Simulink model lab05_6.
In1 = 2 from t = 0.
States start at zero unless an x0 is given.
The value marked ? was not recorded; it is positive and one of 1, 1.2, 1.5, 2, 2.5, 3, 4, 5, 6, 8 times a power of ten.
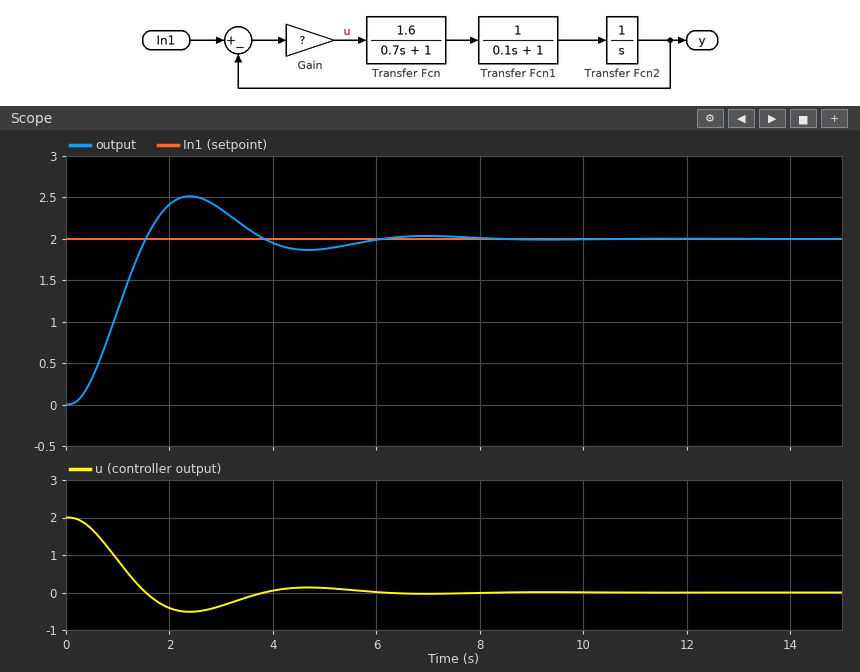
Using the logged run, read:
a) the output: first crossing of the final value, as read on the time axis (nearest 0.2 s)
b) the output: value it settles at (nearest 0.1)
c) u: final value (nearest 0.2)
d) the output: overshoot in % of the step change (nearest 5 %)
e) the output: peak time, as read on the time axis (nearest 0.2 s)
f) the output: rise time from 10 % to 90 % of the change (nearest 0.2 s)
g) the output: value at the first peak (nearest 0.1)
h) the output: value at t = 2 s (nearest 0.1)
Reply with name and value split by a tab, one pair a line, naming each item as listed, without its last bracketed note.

the output: first crossing of the final value, as read on the time axis	1.6 s
the output: value it settles at	2.0
u: final value	0.0
the output: overshoot in % of the step change	25 %
the output: peak time, as read on the time axis	2.4 s
the output: rise time from 10 % to 90 % of the change	1.0 s
the output: value at the first peak	2.5
the output: value at t = 2 s	2.4
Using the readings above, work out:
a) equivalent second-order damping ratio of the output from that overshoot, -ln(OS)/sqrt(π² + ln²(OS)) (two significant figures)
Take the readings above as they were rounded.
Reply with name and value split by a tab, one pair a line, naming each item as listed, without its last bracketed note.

equivalent second-order damping ratio of the output from that overshoot, -ln(OS)/sqrt(π² + ln²(OS))	0.40
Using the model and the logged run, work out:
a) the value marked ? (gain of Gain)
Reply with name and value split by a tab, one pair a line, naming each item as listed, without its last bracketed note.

the value marked ?	1
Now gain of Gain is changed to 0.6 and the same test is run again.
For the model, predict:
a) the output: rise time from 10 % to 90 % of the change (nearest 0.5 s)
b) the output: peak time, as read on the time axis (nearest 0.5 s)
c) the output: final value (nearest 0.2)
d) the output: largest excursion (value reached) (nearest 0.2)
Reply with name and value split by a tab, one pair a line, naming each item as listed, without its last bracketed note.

the output: rise time from 10 % to 90 % of the change	1.5 s
the output: peak time, as read on the time axis	3.5 s
the output: final value	2.0
the output: largest excursion (value reached)	2.2
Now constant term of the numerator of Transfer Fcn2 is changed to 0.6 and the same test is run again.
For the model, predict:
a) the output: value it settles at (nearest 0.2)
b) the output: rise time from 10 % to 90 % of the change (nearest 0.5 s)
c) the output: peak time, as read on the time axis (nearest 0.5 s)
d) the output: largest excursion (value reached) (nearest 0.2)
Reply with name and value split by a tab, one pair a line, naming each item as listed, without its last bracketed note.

the output: value it settles at	2.0
the output: rise time from 10 % to 90 % of the change	1.5 s
the output: peak time, as read on the time axis	3.5 s
the output: largest excursion (value reached)	2.2
